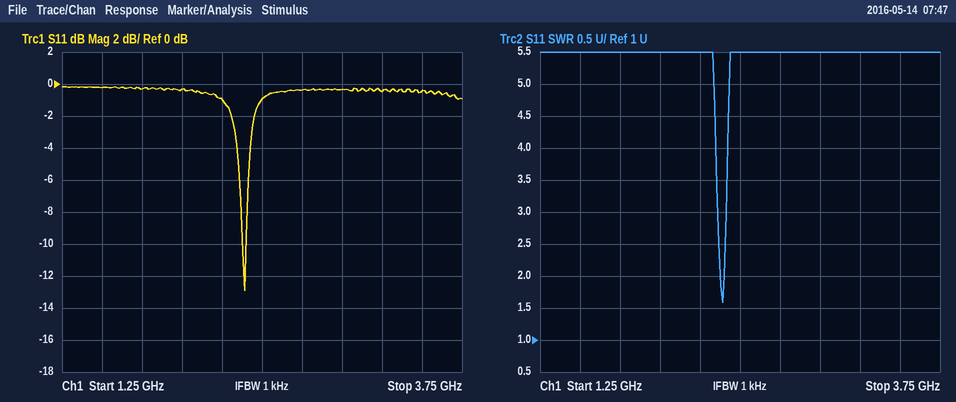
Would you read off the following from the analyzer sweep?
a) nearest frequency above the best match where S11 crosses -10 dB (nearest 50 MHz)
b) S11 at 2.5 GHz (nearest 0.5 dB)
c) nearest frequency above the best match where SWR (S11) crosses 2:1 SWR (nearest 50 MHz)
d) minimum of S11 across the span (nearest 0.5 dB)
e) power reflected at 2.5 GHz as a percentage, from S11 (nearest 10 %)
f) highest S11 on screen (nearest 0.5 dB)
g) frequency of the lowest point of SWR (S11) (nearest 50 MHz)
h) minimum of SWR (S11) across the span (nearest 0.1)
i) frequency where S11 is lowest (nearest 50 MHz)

2.40 GHz
-1.0 dB
2.40 GHz
-13.0 dB
80 %
0.0 dB
2.40 GHz
1.6
2.40 GHz
